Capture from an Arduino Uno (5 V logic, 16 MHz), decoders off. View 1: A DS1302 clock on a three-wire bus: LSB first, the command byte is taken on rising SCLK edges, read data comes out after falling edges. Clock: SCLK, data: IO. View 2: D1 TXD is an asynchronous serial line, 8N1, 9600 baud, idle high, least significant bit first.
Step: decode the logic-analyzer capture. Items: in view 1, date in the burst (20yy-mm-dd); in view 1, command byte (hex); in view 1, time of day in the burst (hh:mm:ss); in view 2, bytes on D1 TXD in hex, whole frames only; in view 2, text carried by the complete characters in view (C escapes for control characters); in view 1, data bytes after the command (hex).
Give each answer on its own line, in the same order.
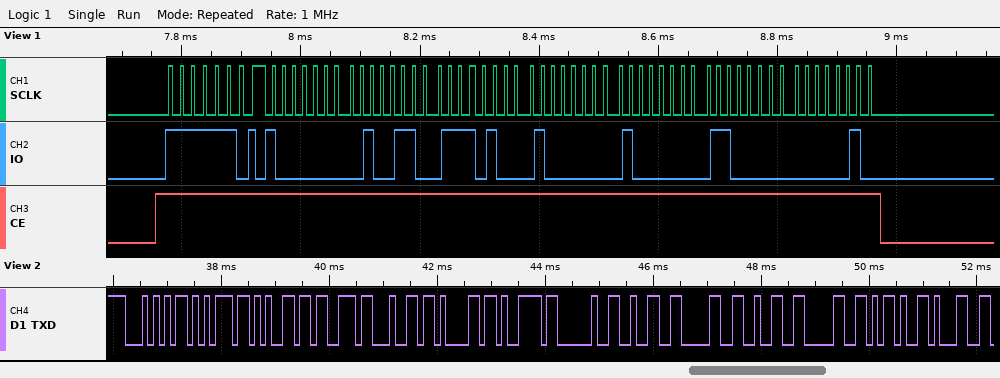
2020-01-01
0xBF
17:32:01
54 75 65 73 64 61 79 20 32 30 32 30 2D 31
"Tuesday 2020-1"
01 32 17 01 01 03 20
